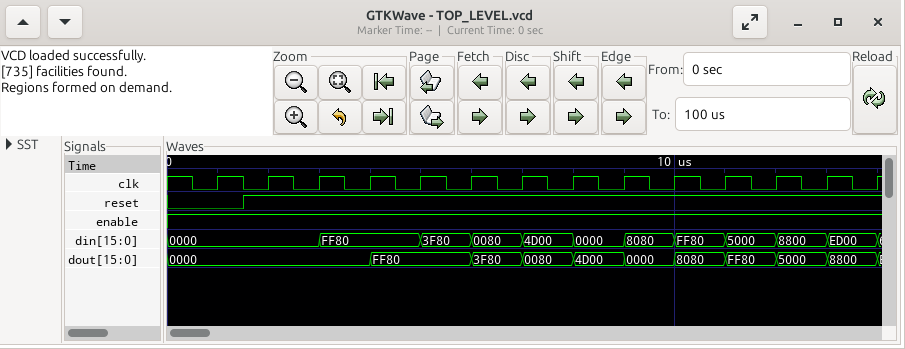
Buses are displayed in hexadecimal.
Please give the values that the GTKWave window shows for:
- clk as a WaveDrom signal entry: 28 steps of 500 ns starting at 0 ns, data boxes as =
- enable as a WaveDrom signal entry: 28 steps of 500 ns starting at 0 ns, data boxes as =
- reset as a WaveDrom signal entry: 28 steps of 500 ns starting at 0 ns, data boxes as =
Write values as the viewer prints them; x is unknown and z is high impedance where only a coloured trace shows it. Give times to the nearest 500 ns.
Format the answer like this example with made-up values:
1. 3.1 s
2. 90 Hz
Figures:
1. {name: 'clk', wave: '1010101010101010101010101010'}
2. {name: 'enable', wave: '1...........................'}
3. {name: 'reset', wave: '0..1........................'}
